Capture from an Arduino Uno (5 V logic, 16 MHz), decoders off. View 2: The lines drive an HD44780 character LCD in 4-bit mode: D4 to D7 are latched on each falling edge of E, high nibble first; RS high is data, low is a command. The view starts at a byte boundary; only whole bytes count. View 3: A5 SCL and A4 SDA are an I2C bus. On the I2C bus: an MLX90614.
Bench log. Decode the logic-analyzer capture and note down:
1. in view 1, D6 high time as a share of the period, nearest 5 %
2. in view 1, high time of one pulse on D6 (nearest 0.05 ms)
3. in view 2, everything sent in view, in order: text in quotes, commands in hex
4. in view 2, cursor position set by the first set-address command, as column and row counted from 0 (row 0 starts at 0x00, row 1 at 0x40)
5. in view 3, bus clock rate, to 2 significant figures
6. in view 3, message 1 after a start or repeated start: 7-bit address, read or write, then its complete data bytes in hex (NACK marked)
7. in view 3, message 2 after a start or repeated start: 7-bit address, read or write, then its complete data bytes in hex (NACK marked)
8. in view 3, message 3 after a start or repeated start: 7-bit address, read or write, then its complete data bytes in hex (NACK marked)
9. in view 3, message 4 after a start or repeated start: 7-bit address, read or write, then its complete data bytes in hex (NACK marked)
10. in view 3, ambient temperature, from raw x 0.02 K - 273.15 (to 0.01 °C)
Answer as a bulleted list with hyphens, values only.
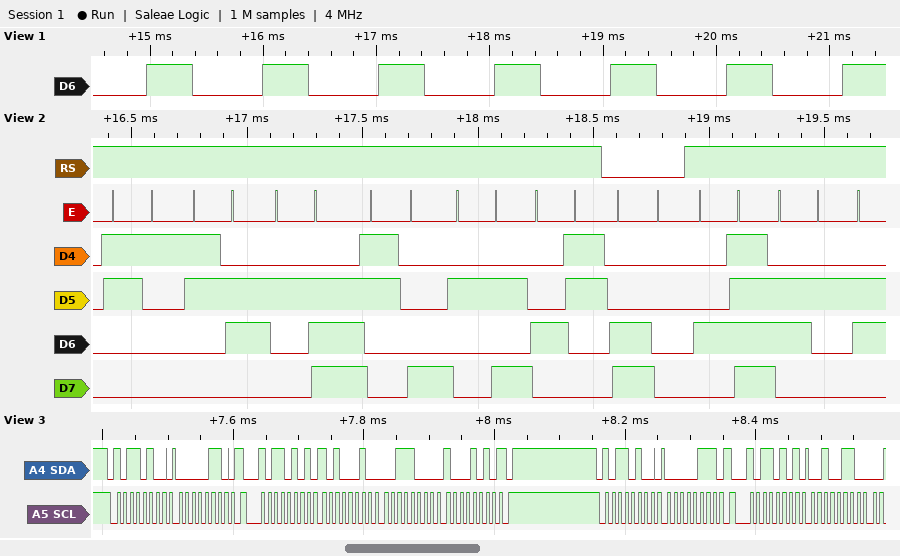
- 40 %
- 0.40 ms
- "16.8*C" 0xC0 "Ob"
- column 0, row 1
- 100 kHz
- 0x5A write: 06
- 0x5A read: A2 38 8A NACK
- 0x5A write: 07
- 0x5A read: 26
- 16.81 °C
